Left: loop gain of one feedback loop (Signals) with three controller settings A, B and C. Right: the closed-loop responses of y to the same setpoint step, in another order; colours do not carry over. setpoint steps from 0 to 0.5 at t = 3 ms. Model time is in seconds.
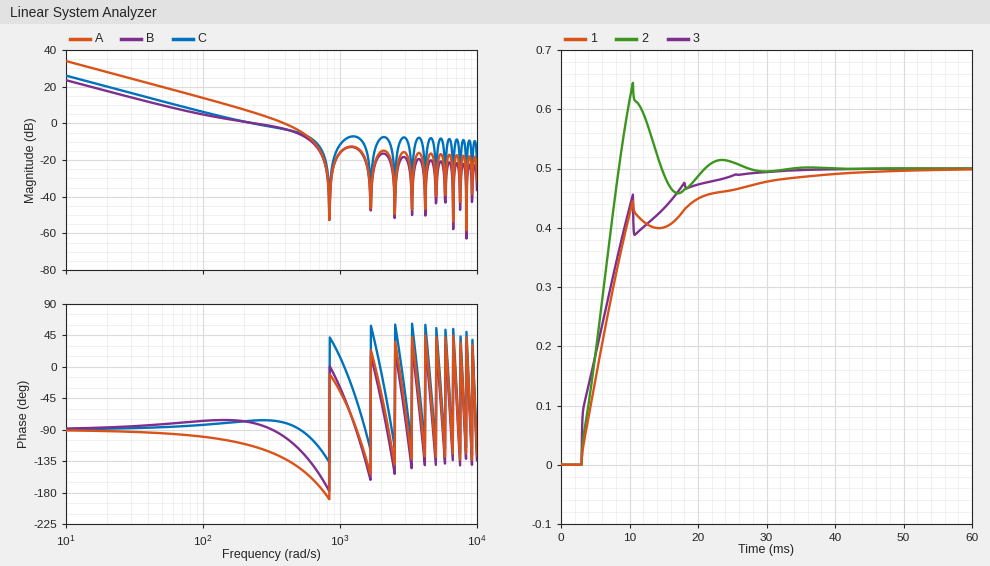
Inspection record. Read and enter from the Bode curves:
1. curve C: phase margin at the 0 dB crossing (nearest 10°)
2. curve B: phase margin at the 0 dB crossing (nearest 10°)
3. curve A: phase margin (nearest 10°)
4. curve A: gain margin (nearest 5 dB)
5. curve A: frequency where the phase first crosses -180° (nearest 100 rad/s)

100°
100°
50°
20 dB
800 rad/s
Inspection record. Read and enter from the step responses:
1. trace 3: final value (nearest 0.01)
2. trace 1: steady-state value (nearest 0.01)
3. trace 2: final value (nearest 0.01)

0.50
0.50
0.50
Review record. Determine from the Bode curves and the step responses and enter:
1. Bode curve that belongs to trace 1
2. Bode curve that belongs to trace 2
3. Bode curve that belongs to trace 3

B
A
C
